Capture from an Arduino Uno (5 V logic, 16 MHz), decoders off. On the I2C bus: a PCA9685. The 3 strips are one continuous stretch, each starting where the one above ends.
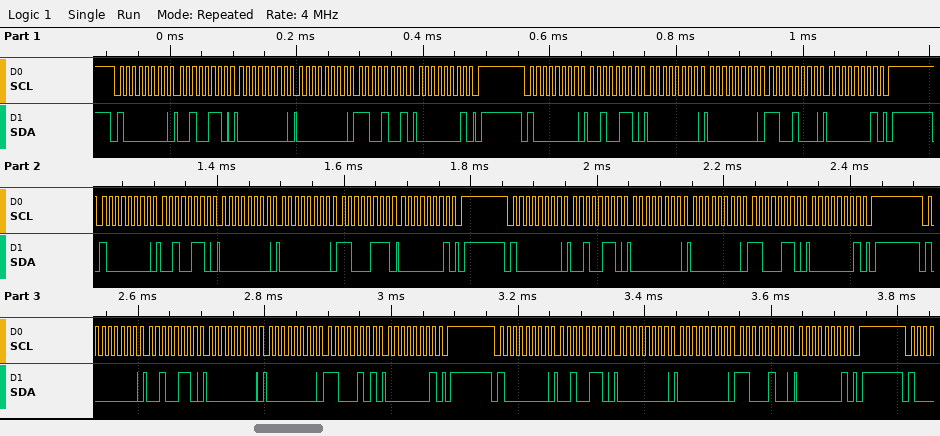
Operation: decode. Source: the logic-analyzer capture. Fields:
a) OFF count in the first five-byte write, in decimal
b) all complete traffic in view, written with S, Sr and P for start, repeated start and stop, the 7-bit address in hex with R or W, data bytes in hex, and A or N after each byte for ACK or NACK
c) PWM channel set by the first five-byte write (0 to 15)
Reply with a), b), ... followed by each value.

a) 457
b) S 40W A 26 A 00 A 00 A C9 A 01 A P S 40W A 26 A 00 A 00 A C8 A 01 A P S 40W A 26 A 00 A 00 A C7 A 01 A P S 40W A 26 A 00 A 00 A C6 A 01 A P S 40W A 26 A 00 A 00 A C5 A 01 A P S 40W A 26 A 00 A 00 A C4 A 01 A P
c) 8
